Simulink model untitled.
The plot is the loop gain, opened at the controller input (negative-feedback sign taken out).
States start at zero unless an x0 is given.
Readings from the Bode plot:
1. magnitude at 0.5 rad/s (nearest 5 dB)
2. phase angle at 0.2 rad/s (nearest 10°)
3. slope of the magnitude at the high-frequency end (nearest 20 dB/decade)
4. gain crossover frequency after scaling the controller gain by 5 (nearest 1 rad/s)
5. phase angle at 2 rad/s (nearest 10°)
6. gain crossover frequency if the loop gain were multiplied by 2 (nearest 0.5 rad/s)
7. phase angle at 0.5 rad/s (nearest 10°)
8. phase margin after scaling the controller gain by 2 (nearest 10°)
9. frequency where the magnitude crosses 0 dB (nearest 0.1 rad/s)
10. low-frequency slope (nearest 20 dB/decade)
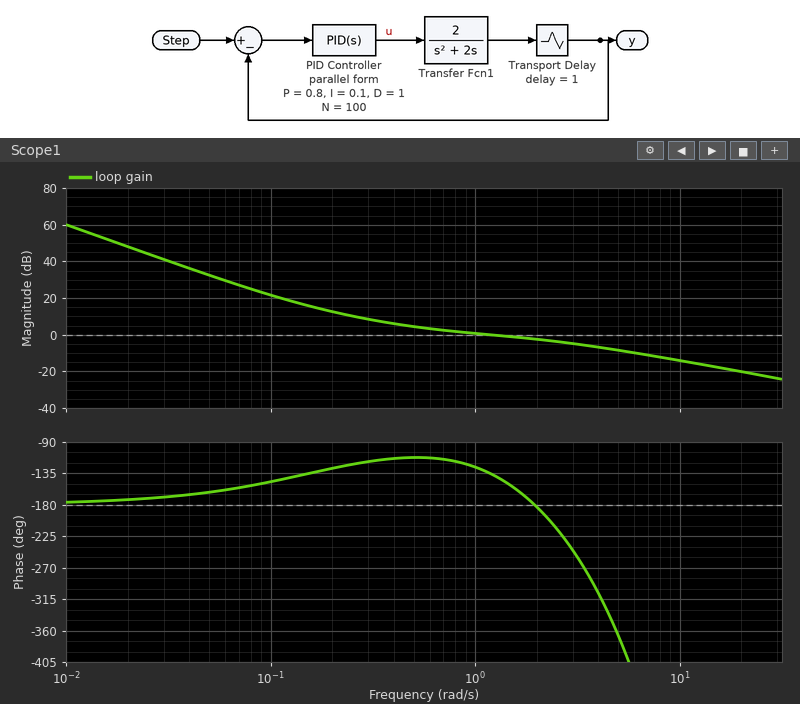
5 dB
-130°
-20 dB/decade
10 rad/s
-180°
3.5 rad/s
-110°
-100°
1.2 rad/s
-40 dB/decade
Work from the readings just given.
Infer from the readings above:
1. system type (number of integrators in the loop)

2
